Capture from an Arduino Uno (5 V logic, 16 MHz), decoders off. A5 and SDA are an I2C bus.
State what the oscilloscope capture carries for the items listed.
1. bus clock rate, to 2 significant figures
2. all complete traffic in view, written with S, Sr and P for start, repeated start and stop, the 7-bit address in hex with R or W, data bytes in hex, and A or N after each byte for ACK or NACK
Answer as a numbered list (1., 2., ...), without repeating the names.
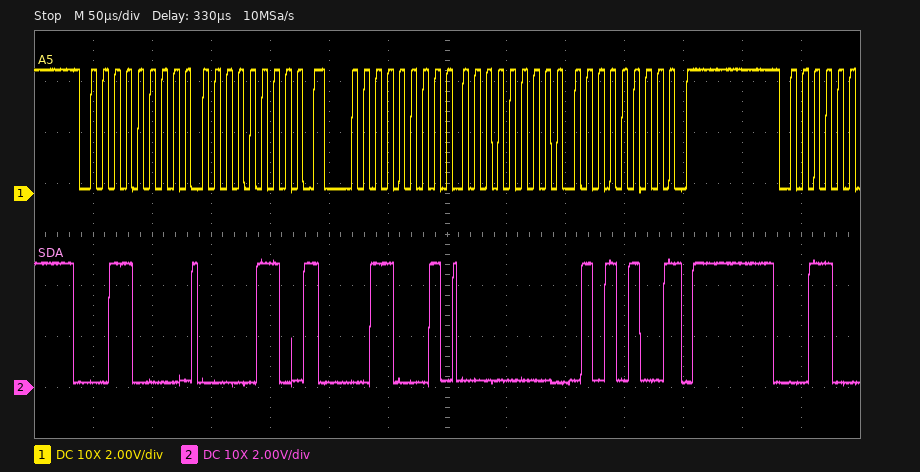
1. 100 kHz
2. S 18W A 06 A Sr 18R A 00 A 54 N P
